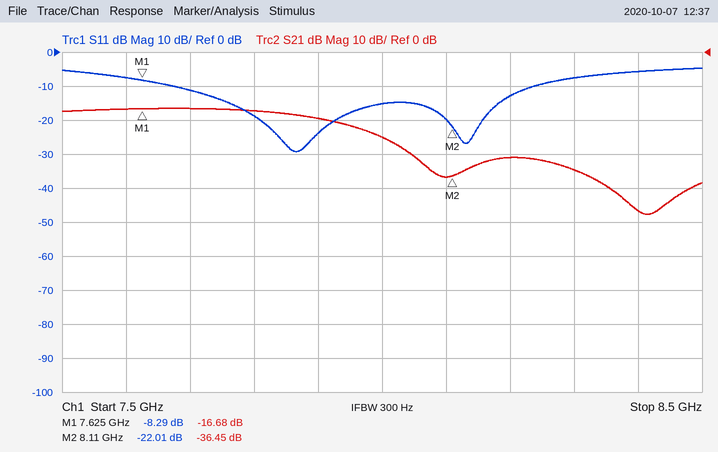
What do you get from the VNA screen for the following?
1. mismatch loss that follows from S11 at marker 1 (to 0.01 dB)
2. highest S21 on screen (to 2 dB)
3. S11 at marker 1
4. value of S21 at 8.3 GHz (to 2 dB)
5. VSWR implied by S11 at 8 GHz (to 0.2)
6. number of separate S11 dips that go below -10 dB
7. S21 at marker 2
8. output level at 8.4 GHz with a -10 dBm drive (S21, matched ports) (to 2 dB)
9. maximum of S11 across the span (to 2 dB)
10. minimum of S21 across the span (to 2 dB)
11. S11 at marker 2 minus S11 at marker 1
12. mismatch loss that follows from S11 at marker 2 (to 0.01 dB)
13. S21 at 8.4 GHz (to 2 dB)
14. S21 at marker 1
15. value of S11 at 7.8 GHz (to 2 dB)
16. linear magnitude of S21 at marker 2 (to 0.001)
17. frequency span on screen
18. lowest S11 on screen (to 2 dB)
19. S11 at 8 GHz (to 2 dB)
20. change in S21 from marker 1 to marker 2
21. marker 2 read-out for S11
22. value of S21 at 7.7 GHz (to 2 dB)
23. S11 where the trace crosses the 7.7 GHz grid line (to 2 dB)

0.70 dB
-16 dB
-8.29 dB
-34 dB
1.4
2
-36.45 dB
-56 dBm
-4 dB
-48 dB
-13.72 dB
0.03 dB
-46 dB
-16.68 dB
-18 dB
0.015
1 GHz
-30 dB
-16 dB
-19.77 dB
-22.01 dB
-16 dB
-12 dB
